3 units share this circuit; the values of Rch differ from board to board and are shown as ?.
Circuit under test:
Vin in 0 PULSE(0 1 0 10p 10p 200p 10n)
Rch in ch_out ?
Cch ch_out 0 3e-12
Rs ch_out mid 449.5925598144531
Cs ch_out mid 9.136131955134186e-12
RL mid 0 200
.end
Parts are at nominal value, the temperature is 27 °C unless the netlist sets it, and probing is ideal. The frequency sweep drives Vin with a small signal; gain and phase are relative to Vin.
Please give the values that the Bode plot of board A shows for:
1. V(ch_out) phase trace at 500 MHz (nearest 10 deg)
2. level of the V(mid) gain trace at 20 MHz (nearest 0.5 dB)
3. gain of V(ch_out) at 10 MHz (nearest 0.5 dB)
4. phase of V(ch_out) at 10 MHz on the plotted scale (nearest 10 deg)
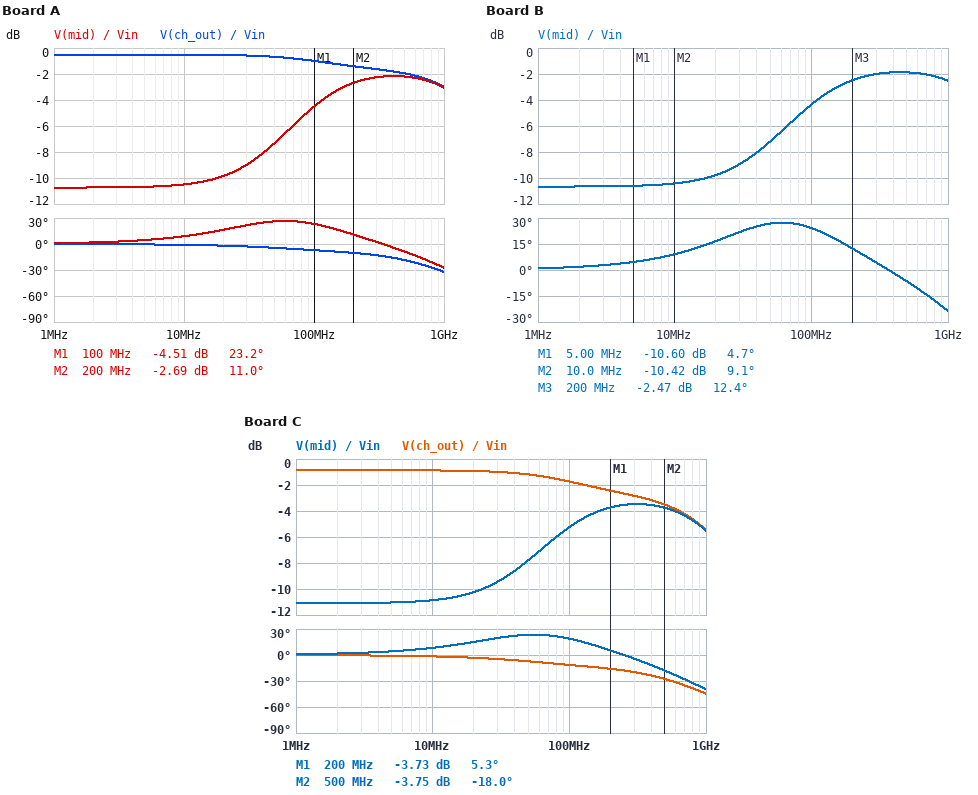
-20 deg
-10.0 dB
-0.5 dB
0 deg
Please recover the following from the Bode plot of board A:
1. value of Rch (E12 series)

39 Ω
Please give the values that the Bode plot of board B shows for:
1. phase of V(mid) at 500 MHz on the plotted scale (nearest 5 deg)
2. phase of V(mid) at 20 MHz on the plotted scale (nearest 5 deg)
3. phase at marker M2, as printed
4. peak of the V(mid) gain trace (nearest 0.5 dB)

-5 deg
15 deg
9.1 deg
-2.0 dB
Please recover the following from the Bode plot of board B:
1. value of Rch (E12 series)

33 Ω
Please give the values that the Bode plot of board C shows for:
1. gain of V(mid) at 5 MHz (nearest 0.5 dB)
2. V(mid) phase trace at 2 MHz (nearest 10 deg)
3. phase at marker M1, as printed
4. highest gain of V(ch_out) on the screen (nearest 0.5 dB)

-11.0 dB
0 deg
5.3 deg
-1.0 dB
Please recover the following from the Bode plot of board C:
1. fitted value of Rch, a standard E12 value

68 Ω
